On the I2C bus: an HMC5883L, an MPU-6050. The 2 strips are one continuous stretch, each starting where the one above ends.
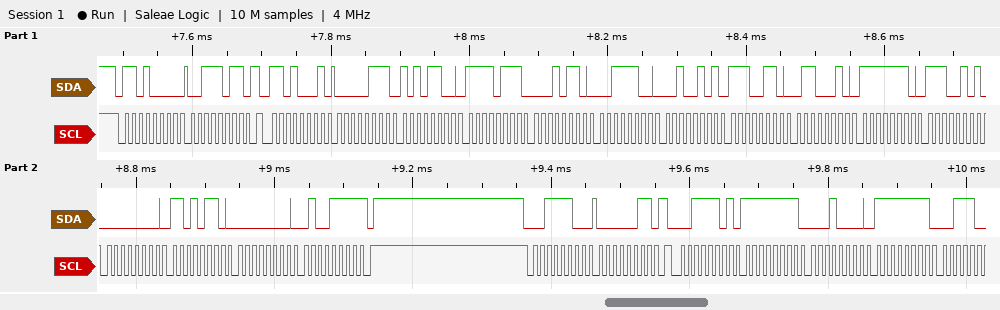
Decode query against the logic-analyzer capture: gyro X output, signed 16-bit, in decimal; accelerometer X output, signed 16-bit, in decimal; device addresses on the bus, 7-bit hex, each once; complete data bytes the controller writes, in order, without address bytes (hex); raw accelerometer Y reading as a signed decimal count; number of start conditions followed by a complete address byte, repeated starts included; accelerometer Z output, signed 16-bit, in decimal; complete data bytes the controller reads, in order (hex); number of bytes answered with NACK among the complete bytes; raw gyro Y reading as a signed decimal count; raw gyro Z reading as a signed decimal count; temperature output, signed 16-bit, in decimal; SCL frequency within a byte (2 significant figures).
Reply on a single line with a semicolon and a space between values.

-283; 1964; 0x68 0x1E; 3B 03; -2282; 4; 15397; 07 AC F7 16 3C 25 E6 62 FE E5 00 D6 00 4F FF 10 FF; 1; 214; 79; -6558; 100 kHz
